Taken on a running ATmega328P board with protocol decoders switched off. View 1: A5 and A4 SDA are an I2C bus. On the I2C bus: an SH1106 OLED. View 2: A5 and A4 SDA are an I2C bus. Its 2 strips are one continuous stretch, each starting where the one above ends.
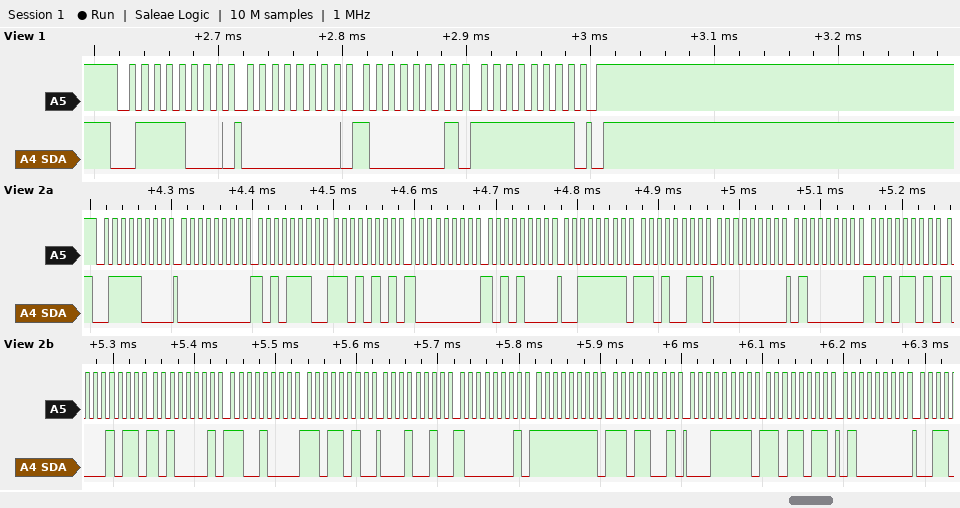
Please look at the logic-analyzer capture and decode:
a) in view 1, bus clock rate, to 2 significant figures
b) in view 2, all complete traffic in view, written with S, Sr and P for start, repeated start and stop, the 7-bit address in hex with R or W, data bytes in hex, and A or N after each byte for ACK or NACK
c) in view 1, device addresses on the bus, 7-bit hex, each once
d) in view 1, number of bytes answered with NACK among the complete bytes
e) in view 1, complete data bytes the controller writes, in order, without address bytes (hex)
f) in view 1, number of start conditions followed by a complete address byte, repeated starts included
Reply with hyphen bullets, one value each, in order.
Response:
- 100 kHz
- S 3CW A 00 A AE A D5 A 80 A A8 A 3F A D3 A 00 A 40 A AD A 8B A A1 A C8 A DA A 12 A 81 A FF A D9 A 1F A DB A 40 A
- 0x3C
- 0
- 00 81 FF
- 1
